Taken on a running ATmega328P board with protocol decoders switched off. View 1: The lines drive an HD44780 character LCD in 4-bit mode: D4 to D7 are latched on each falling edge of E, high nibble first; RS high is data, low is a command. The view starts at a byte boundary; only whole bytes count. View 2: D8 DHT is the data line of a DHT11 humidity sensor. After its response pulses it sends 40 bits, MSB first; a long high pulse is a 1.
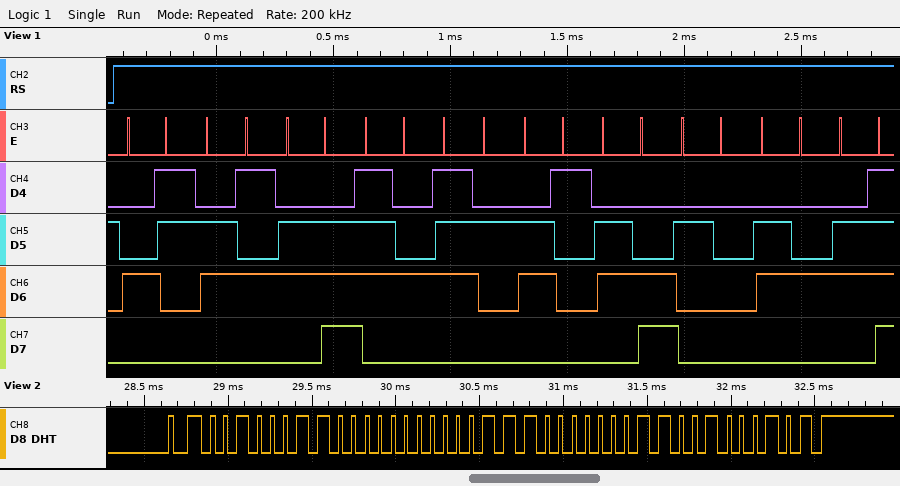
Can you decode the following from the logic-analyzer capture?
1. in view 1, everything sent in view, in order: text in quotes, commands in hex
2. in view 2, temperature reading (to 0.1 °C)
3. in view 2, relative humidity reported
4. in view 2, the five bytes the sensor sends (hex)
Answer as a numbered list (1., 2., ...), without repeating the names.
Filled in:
1. "Central do"
2. 28.6 °C
3. 35 %
4. 23 00 1C 06 45
